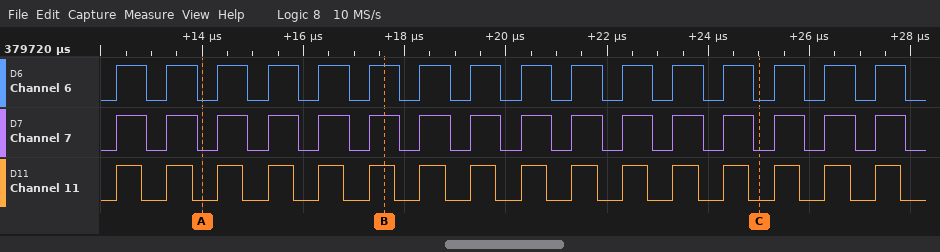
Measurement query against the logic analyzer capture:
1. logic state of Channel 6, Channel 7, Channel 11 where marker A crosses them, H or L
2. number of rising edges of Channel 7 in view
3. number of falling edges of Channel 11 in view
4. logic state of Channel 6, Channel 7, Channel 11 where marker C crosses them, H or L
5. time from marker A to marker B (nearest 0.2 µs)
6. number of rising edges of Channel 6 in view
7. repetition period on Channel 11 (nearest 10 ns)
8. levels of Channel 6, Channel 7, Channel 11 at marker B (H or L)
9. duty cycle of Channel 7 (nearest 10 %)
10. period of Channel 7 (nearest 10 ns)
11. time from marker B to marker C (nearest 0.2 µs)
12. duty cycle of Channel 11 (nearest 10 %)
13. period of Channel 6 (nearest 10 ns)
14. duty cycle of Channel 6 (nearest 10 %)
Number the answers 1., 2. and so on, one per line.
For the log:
1. Channel 6=L, Channel 7=L, Channel 11=L
2. 16
3. 16
4. Channel 6=L, Channel 7=L, Channel 11=L
5. 3.6 µs
6. 16
7. 1000 ns
8. Channel 6=H, Channel 7=H, Channel 11=H
9. 60 %
10. 1000 ns
11. 7.4 µs
12. 50 %
13. 1000 ns
14. 60 %
